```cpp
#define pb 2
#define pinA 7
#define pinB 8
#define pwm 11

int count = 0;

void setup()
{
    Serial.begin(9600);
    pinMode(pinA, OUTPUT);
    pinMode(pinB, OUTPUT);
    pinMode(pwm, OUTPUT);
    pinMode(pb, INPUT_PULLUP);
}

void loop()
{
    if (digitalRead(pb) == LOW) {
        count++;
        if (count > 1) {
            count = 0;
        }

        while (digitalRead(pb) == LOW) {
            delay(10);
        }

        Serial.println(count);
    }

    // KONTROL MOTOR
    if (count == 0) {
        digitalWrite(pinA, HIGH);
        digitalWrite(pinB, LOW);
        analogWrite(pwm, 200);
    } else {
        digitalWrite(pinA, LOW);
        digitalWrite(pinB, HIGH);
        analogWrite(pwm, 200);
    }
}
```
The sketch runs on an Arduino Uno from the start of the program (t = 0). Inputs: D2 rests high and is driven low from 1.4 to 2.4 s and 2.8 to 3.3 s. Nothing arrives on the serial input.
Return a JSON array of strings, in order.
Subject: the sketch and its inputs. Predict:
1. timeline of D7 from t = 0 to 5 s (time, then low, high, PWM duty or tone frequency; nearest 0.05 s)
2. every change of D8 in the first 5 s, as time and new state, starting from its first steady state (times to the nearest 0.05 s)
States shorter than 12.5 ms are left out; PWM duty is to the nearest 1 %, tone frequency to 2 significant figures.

["0 s high; 2.4 s low; 3.3 s high", "0 s low; 2.4 s high; 3.3 s low"]
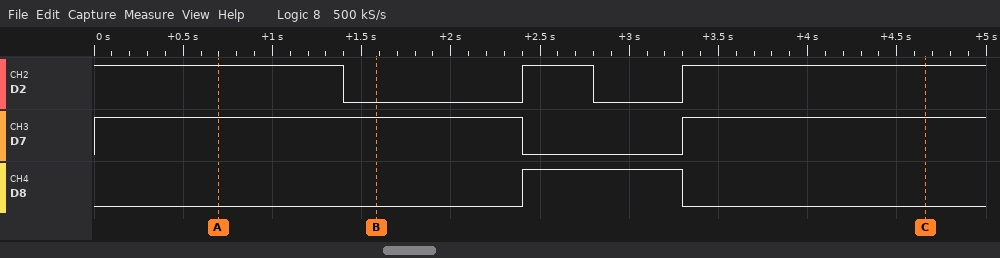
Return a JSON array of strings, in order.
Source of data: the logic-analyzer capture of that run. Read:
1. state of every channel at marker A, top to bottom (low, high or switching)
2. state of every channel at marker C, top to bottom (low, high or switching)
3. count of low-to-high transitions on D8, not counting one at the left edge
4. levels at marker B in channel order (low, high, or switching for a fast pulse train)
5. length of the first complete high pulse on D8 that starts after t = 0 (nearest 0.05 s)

["D2 high, D7 high, D8 low", "D2 high, D7 high, D8 low", "1", "D2 low, D7 high, D8 low", "0.90 s"]
